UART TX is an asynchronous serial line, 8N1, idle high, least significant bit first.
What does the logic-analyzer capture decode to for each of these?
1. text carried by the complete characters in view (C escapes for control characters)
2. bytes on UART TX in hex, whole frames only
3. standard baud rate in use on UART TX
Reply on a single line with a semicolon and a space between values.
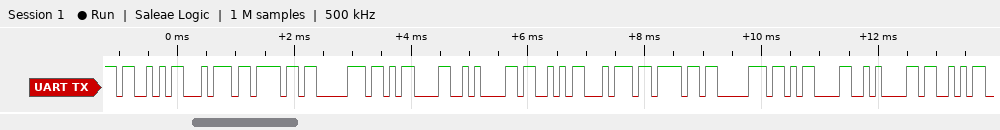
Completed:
"Stop\r\nStop\r\nS"; 53 74 6F 70 0D 0A 53 74 6F 70 0D 0A 53; 9600 baud
